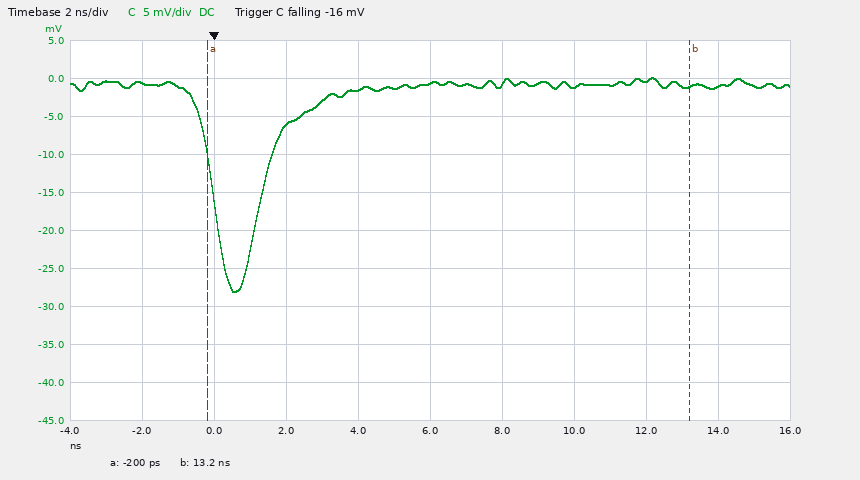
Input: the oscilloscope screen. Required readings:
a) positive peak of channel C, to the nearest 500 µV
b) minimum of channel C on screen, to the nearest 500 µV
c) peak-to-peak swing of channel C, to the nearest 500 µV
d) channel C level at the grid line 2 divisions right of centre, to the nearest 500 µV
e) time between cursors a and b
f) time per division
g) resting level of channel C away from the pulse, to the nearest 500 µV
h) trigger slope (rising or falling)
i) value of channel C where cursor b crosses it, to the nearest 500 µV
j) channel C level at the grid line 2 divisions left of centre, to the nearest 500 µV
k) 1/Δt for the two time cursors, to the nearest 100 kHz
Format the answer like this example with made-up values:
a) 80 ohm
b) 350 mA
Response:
a) 0.0 mV
b) -28.0 mV
c) 28.0 mV
d) -1.0 mV
e) 13.4 ns
f) 2 ns
g) -1.0 mV
h) falling
i) -1.0 mV
j) -6.0 mV
k) 74.6 MHz
